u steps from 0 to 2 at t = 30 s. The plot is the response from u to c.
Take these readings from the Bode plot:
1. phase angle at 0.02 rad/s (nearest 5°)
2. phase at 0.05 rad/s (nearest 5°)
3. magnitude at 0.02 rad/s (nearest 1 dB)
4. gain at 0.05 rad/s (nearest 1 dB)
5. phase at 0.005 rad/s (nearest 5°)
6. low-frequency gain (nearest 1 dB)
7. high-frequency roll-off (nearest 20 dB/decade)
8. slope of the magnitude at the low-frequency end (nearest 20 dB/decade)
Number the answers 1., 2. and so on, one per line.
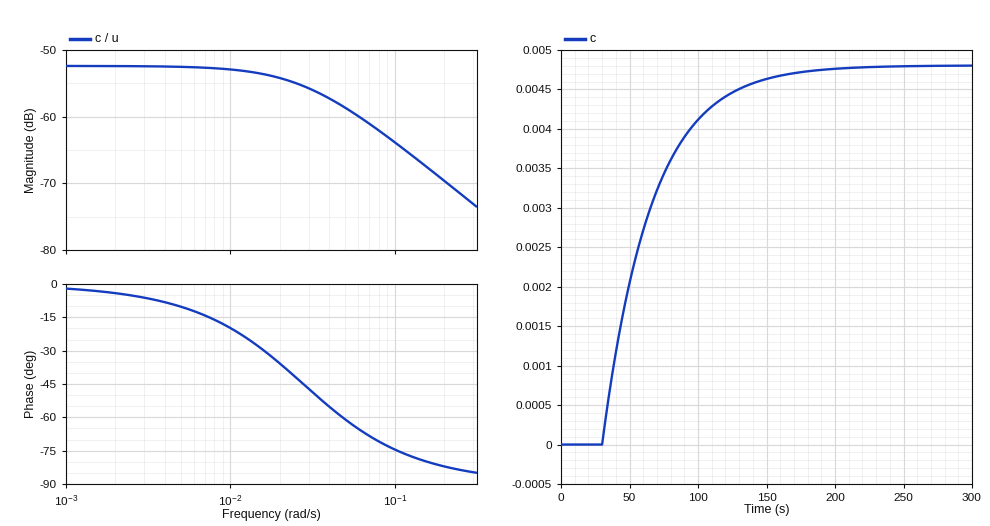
1. -35°
2. -60°
3. -54 dB
4. -59 dB
5. -10°
6. -52 dB
7. -20 dB/decade
8. 0 dB/decade
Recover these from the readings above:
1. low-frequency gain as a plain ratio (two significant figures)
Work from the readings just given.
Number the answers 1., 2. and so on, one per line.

1. 0.0025
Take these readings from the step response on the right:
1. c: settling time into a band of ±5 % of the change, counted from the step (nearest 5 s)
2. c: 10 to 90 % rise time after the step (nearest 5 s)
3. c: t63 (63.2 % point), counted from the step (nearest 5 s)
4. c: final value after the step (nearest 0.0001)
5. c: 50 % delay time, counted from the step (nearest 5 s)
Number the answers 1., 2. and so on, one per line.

1. 110 s
2. 80 s
3. 35 s
4. 0.0048
5. 25 s
